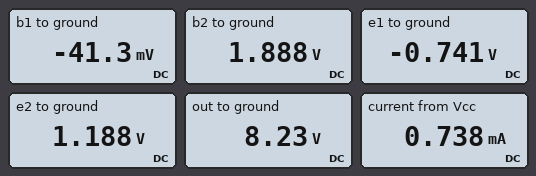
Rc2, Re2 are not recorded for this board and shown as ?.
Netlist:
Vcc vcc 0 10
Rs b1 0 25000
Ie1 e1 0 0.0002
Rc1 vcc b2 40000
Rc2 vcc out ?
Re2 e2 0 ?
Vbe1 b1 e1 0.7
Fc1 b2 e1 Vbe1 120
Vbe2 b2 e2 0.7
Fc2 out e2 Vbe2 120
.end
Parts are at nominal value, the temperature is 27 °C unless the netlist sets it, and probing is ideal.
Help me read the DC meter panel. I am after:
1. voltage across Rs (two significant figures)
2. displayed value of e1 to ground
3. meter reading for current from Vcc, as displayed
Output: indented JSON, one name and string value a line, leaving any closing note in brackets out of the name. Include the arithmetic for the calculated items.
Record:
{
  "voltage across Rs": "0 V - (-41.3 mV) = 41 mV",
  "displayed value of e1 to ground": "-0.741 V",
  "meter reading for current from Vcc, as displayed": "0.738 mA"
}
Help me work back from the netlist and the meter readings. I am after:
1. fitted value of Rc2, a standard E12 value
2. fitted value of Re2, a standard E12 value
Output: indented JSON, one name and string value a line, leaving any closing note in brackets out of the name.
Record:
{
  "fitted value of Rc2, a standard E12 value": "3.3 kΩ",
  "fitted value of Re2, a standard E12 value": "2.2 kΩ"
}
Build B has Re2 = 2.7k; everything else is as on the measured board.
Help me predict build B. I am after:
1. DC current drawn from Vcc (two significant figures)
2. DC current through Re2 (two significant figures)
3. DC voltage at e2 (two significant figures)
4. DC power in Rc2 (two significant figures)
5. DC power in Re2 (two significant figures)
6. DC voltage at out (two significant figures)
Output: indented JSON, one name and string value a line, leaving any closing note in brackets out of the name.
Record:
{
  "DC current drawn from Vcc": "650 µA",
  "DC current through Re2": "450 µA",
  "DC voltage at e2": "1.2 V",
  "DC power in Rc2": "660 µW",
  "DC power in Re2": "550 µW",
  "DC voltage at out": "8.5 V"
}
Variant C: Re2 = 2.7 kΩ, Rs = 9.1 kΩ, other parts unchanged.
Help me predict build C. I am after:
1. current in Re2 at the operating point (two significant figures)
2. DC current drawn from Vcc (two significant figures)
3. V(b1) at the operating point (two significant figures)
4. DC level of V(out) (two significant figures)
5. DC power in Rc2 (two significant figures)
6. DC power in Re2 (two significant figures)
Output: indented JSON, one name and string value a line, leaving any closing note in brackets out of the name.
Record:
{
  "current in Re2 at the operating point": "450 µA",
  "DC current drawn from Vcc": "650 µA",
  "V(b1) at the operating point": "-15 mV",
  "DC level of V(out)": "8.5 V",
  "DC power in Rc2": "660 µW",
  "DC power in Re2": "550 µW"
}
